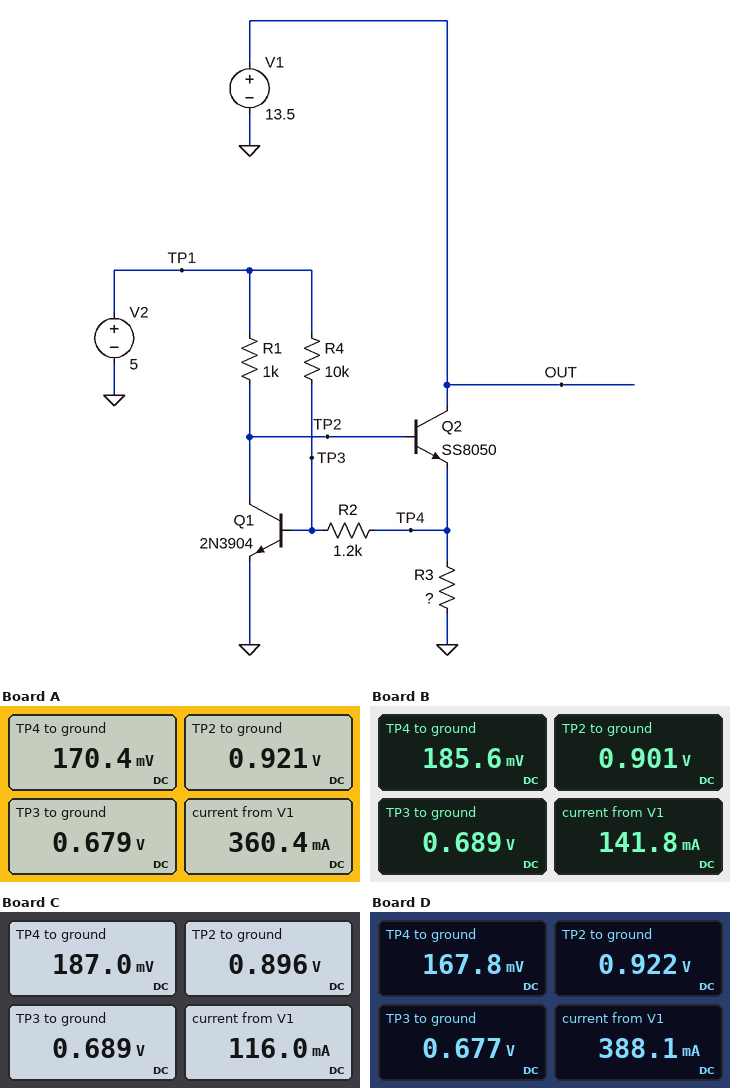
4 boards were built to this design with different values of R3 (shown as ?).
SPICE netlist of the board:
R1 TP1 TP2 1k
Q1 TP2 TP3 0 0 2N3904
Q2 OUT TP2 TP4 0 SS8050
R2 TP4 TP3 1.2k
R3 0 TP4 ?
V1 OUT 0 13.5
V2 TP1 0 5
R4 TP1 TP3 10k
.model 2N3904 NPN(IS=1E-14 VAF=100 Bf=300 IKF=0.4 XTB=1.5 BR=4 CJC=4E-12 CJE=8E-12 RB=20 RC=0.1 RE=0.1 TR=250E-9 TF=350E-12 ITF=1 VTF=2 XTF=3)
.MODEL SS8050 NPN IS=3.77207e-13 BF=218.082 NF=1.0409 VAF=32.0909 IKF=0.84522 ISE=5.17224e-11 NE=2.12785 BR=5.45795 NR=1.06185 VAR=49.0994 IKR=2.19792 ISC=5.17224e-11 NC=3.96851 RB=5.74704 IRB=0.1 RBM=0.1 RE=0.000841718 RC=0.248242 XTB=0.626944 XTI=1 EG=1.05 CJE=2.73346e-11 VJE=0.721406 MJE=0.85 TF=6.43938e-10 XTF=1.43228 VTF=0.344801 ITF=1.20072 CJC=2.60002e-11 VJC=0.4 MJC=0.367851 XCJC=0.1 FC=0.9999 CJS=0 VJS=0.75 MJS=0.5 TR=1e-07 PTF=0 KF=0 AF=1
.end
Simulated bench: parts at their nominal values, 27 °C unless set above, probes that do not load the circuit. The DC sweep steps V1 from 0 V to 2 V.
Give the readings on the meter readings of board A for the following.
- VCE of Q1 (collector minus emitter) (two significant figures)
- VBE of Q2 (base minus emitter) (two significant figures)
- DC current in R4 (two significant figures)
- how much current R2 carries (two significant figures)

920 mV
750 mV
430 µA
420 µA
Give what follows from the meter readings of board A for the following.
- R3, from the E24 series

0.47 Ω
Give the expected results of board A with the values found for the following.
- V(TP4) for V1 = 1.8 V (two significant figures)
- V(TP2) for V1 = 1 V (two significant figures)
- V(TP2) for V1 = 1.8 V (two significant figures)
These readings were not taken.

160 mV
920 mV
920 mV
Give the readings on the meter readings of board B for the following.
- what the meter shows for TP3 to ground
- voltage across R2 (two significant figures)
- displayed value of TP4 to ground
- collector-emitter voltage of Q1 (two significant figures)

0.689 V
500 mV
185.6 mV
900 mV
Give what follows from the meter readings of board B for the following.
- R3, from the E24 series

1.3 Ω
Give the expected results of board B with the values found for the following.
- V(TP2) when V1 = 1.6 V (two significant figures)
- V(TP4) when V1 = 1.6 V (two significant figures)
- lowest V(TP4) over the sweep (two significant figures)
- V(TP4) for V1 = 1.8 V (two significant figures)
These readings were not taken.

910 mV
180 mV
7.4 mV
180 mV
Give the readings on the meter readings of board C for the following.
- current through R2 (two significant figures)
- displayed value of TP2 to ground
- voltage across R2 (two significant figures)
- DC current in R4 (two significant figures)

420 µA
0.896 V
500 mV
430 µA
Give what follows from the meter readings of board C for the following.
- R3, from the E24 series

1.6 Ω
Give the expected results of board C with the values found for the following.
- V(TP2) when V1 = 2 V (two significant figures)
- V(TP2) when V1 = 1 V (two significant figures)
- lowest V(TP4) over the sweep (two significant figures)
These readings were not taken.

900 mV
900 mV
8.1 mV
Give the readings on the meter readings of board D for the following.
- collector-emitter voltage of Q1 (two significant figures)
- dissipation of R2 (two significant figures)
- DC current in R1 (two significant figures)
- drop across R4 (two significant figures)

920 mV
220 µW
4.1 mA
4.3 V
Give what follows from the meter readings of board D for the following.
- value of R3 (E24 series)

0.43 Ω
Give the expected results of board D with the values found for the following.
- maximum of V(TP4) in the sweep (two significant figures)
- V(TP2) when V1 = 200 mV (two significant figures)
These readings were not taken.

160 mV
840 mV
